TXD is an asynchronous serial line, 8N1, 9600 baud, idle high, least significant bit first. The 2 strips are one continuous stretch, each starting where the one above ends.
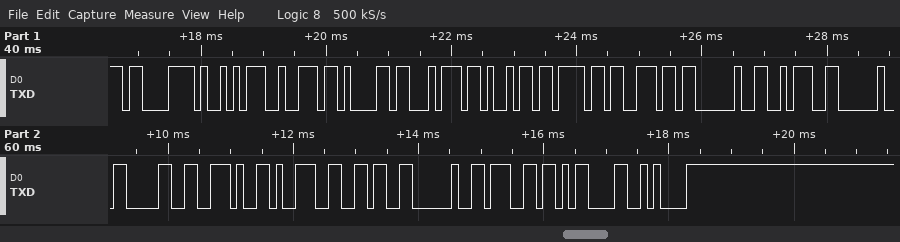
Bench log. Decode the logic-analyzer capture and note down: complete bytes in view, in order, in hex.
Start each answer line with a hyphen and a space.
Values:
- C3 A9 72 61 74 69 6F 6E 20 3A 20 30 2E 39 36 20 67 0D 0A
